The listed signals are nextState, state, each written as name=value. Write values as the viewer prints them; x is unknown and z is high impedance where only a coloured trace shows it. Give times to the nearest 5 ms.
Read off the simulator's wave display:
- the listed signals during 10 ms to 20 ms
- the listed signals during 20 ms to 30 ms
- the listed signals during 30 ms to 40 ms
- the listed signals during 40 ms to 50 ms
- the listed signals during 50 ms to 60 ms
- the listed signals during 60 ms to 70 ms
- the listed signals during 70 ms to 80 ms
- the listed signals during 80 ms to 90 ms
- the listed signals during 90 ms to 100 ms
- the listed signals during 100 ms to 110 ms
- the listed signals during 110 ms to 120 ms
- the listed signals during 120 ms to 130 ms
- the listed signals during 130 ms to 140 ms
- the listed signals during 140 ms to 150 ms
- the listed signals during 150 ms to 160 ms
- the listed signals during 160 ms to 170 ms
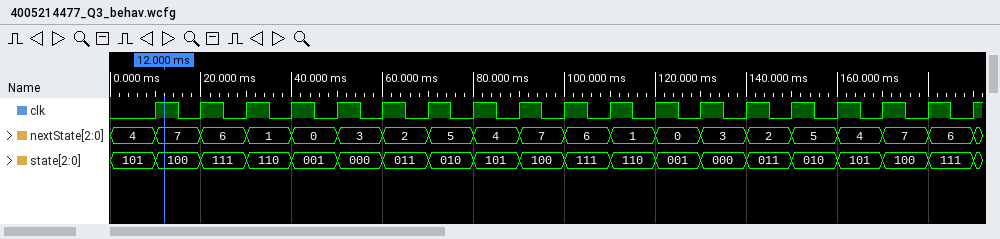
nextState=7, state=100
nextState=6, state=111
nextState=1, state=110
nextState=0, state=001
nextState=3, state=000
nextState=2, state=011
nextState=5, state=010
nextState=4, state=101
nextState=7, state=100
nextState=6, state=111
nextState=1, state=110
nextState=0, state=001
nextState=3, state=000
nextState=2, state=011
nextState=5, state=010
nextState=4, state=101
